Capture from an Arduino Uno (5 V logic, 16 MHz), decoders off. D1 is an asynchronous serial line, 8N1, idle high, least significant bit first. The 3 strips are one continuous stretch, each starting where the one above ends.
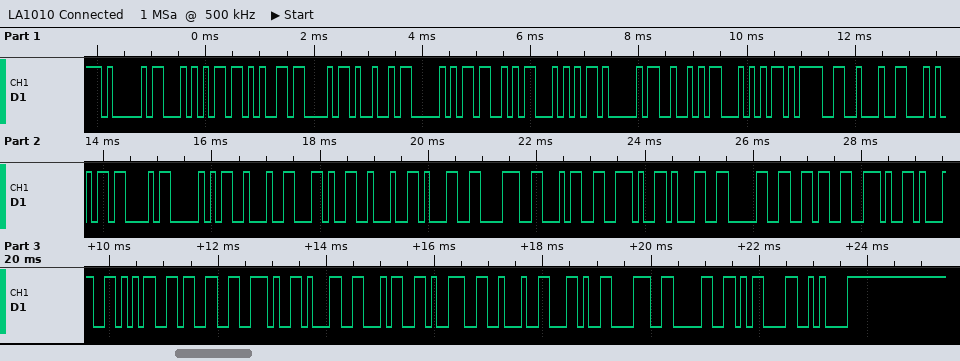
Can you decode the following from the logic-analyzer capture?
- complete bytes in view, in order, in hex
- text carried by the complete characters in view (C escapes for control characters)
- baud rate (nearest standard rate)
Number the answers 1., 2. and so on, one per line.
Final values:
1. 0x41 0x54 0x2B 0x43 0x49 0x50 0x53 0x54 0x41 0x52 0x54 0x3D 0x22 0x54 0x43 0x50 0x22 0x2C 0x22 0x31 0x38 0x34 0x2E 0x31 0x30 0x36 0x2E 0x31 0x35 0x33 0x2E 0x31 0x34 0x39 0x22 0x2C 0x38 0x30 0x0D 0x0A
2. "AT+CIPSTART=\"TCP\",\"184.106.153.149\",80\r\n"
3. 9600 baud
